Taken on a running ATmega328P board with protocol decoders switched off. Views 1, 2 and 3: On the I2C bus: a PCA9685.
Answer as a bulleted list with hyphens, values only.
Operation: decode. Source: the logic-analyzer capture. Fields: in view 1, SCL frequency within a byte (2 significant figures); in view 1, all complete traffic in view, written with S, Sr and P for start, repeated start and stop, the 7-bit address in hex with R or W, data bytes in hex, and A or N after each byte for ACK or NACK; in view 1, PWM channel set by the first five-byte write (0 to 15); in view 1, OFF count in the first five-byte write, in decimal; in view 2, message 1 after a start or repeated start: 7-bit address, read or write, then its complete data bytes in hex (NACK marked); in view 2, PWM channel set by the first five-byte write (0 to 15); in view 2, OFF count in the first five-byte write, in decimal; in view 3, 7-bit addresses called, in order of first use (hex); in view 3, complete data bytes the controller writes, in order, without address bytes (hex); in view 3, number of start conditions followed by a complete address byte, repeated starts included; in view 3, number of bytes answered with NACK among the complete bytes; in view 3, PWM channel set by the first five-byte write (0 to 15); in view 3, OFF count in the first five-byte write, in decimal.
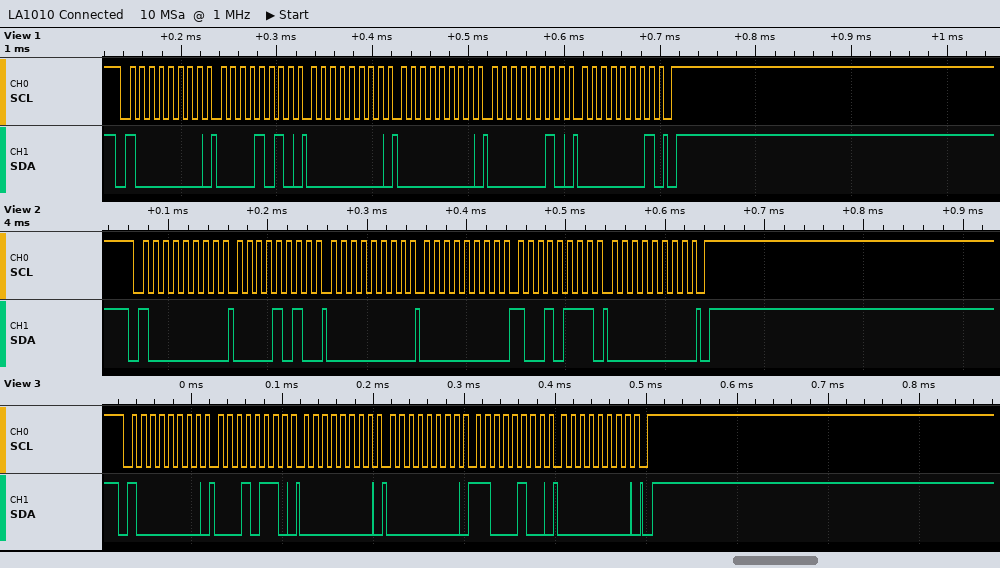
- 100 kHz
- S 40W A 0A A 00 A 00 A 02 A 01 A P
- 1
- 258
- 0x40 write: 0A 00 00 97 00
- 1
- 151
- 0x40
- 16 00 00 C4 00
- 1
- 0
- 4
- 196
